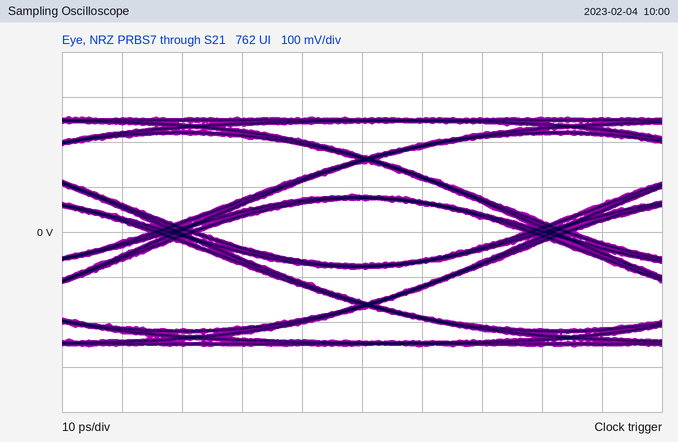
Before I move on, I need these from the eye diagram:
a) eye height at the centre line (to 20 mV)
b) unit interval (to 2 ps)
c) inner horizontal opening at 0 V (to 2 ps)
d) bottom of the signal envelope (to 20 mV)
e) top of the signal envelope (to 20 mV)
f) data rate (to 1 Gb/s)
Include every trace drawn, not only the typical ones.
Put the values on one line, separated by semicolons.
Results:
140 mV; 62 ps; 54 ps; -260 mV; 260 mV; 16 Gb/s
